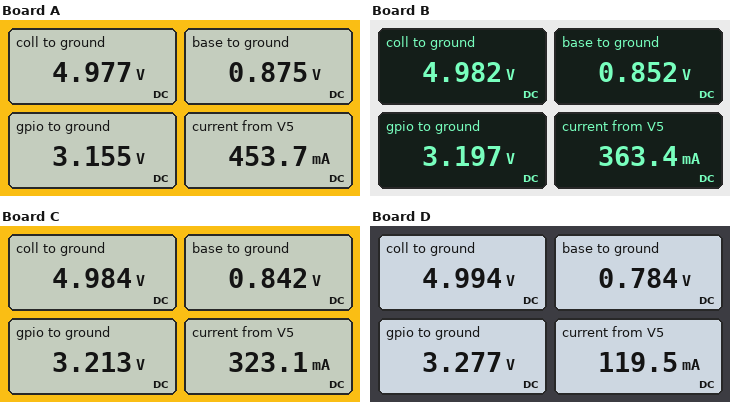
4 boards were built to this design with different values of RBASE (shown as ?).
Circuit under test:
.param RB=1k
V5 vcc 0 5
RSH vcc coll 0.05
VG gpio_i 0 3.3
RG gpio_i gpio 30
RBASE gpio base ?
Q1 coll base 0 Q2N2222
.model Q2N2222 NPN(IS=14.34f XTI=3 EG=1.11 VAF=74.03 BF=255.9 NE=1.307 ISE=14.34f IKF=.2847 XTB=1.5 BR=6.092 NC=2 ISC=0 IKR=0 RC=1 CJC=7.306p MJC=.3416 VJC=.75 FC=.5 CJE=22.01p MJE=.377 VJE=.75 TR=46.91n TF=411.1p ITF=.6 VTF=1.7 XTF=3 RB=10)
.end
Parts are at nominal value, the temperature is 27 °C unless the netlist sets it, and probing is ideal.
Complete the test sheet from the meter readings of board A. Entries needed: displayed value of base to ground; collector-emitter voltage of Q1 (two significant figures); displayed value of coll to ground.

0.875 V
5.0 V
4.977 V
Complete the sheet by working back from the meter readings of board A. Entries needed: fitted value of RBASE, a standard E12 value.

470 Ω
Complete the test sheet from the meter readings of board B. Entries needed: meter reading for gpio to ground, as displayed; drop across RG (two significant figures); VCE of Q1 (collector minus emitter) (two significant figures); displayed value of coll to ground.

3.197 V
100 mV
5.0 V
4.982 V
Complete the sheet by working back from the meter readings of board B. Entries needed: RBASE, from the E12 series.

680 Ω
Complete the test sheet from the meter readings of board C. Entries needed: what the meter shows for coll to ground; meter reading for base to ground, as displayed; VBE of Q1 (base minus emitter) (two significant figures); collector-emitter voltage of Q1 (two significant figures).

4.984 V
0.842 V
840 mV
5.0 V
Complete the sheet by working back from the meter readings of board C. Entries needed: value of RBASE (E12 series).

820 Ω
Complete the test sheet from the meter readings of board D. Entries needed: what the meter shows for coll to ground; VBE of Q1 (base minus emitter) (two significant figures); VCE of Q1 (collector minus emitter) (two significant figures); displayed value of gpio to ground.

4.994 V
780 mV
5.0 V
3.277 V
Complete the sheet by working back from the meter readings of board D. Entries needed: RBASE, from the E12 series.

3.3 kΩ
